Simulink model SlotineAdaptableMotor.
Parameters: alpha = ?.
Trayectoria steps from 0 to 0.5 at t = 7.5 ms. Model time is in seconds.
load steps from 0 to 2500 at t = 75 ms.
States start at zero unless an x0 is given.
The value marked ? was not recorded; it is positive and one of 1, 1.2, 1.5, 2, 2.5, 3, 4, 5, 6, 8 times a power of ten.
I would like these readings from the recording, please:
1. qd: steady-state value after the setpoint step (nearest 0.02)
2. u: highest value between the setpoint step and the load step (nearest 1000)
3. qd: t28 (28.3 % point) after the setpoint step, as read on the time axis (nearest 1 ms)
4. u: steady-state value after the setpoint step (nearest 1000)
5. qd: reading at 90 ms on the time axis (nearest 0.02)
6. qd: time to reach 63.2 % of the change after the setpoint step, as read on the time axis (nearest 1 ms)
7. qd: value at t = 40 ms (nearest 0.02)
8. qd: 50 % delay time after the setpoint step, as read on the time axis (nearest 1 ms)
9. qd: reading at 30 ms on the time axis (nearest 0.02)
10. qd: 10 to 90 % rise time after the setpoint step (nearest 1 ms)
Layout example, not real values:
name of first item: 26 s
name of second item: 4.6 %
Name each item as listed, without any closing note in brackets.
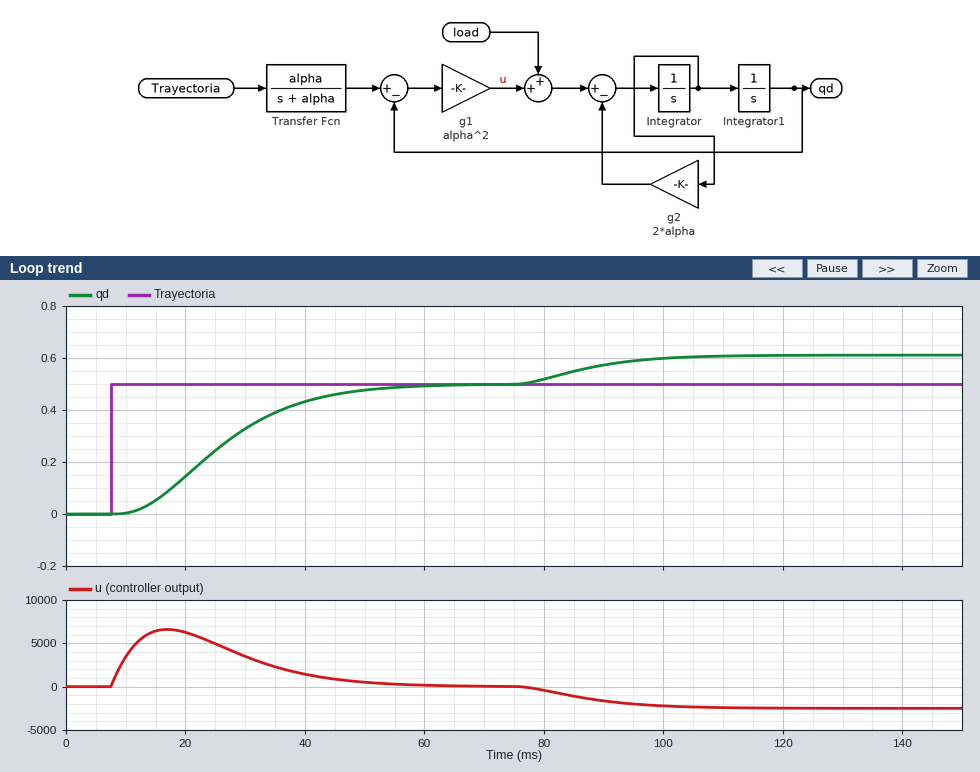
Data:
qd: steady-state value after the setpoint step: 0.50
u: highest value between the setpoint step and the load step: 7000
qd: t28 (28.3 % point) after the setpoint step, as read on the time axis: 20 ms
u: steady-state value after the setpoint step: 0
qd: reading at 90 ms on the time axis: 0.58
qd: time to reach 63.2 % of the change after the setpoint step, as read on the time axis: 29 ms
qd: value at t = 40 ms: 0.44
qd: 50 % delay time after the setpoint step, as read on the time axis: 25 ms
qd: reading at 30 ms on the time axis: 0.32
qd: 10 to 90 % rise time after the setpoint step: 28 ms
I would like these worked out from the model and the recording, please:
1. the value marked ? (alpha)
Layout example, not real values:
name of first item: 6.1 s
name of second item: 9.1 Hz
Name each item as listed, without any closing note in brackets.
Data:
the value marked ?: 150
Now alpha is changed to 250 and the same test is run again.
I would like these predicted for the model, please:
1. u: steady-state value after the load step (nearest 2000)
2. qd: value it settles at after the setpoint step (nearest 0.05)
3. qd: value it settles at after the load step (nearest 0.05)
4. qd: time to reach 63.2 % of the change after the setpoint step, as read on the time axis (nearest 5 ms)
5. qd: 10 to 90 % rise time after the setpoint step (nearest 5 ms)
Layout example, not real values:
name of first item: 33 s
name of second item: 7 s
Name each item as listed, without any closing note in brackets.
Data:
u: steady-state value after the load step: -2000
qd: value it settles at after the setpoint step: 0.50
qd: value it settles at after the load step: 0.55
qd: time to reach 63.2 % of the change after the setpoint step, as read on the time axis: 20 ms
qd: 10 to 90 % rise time after the setpoint step: 15 ms
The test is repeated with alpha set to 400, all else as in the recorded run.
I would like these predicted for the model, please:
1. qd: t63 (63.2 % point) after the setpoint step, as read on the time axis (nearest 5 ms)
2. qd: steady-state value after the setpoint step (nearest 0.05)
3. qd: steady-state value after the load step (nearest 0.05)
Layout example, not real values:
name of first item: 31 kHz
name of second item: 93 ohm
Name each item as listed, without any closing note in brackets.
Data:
qd: t63 (63.2 % point) after the setpoint step, as read on the time axis: 15 ms
qd: steady-state value after the setpoint step: 0.50
qd: steady-state value after the load step: 0.50
